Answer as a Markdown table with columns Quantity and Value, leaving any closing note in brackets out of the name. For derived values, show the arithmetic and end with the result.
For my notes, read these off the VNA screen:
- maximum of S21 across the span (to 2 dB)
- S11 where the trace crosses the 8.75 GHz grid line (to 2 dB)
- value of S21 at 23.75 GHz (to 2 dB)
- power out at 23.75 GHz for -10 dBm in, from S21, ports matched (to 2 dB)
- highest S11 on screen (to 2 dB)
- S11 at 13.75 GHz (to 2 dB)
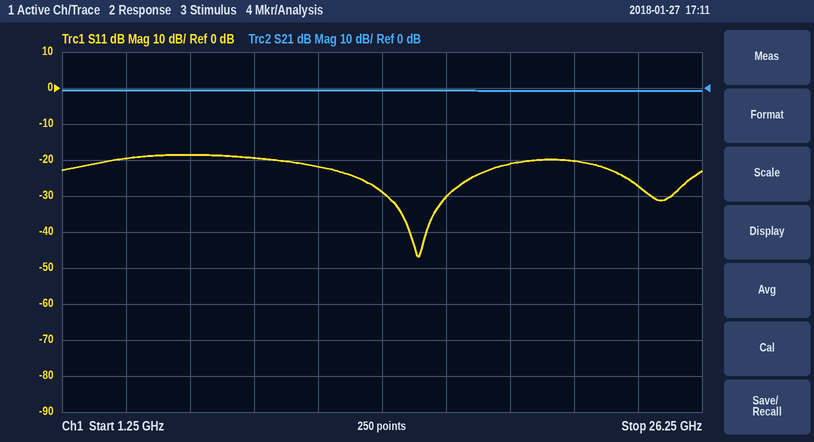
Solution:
| Quantity | Value |
|---|---|
| maximum of S21 across the span | 0 dB |
| S11 where the trace crosses the 8.75 GHz grid line | -20 dB |
| value of S21 at 23.75 GHz | 0 dB |
| power out at 23.75 GHz for -10 dBm in, from S21, ports matched | -10 dBm + (0 dB) = -10 dBm |
| highest S11 on screen | -18 dB |
| S11 at 13.75 GHz | -28 dB |
